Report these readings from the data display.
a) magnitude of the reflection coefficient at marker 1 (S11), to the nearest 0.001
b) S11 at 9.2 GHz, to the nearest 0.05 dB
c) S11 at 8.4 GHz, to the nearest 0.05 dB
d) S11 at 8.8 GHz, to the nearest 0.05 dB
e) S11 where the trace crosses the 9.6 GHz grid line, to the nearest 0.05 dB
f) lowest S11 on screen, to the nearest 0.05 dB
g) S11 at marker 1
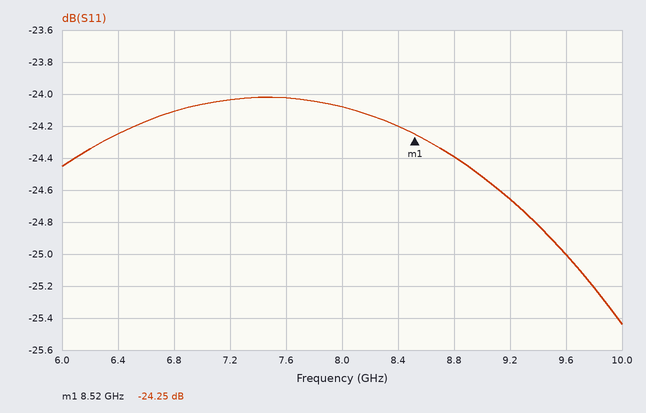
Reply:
0.061
-24.65 dB
-24.20 dB
-24.40 dB
-25.00 dB
-25.45 dB
-24.25 dB
